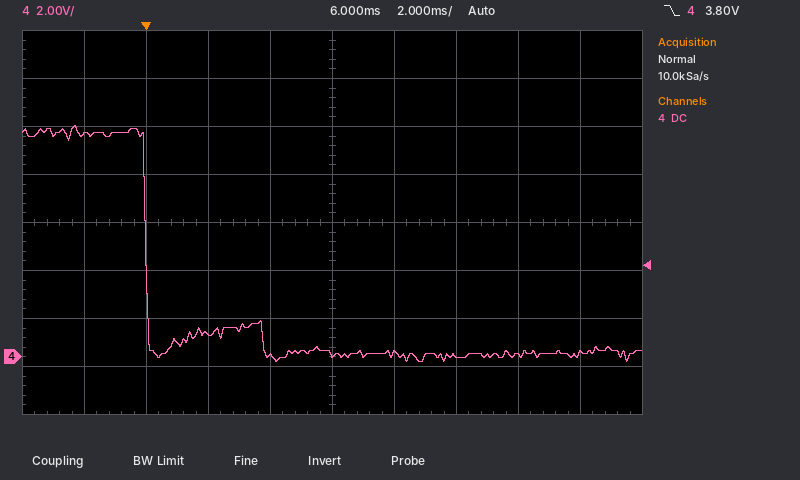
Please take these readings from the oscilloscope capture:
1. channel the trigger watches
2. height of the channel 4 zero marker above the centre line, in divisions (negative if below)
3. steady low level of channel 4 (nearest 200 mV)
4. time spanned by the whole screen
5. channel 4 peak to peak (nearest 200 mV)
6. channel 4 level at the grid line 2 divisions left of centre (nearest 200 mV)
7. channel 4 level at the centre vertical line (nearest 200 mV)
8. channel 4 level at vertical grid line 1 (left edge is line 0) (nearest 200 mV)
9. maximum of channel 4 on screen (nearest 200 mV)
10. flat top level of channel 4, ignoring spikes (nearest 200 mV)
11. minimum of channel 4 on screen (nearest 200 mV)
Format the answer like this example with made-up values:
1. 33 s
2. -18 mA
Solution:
1. channel 4
2. -2.8 div
3. 200 mV
4. 20 ms
5. 9.8 V
6. 1.0 V
7. 200 mV
8. 9.2 V
9. 9.6 V
10. 9.4 V
11. -200 mV
